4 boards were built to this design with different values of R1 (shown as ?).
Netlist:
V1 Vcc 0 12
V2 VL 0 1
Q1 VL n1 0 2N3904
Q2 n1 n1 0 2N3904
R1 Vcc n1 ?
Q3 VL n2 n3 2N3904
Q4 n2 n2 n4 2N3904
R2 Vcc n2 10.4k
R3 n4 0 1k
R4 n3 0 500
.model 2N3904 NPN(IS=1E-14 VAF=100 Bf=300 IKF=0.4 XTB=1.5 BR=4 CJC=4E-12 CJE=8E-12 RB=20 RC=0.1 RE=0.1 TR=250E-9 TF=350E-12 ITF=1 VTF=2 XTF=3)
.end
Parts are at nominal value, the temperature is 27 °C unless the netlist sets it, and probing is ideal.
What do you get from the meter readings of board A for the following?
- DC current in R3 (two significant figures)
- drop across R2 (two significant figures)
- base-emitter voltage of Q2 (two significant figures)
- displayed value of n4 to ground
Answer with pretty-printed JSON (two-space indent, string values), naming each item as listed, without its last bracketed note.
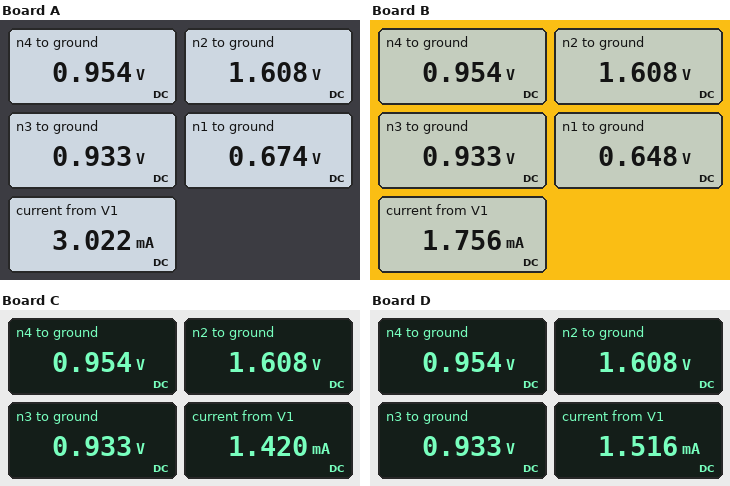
{
  "DC current in R3": "950 µA",
  "drop across R2": "10 V",
  "base-emitter voltage of Q2": "670 mV",
  "displayed value of n4 to ground": "0.954 V"
}
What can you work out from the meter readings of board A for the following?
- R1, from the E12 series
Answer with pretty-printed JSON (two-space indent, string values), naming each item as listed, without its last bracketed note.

{
  "R1, from the E12 series": "5.6 kΩ"
}
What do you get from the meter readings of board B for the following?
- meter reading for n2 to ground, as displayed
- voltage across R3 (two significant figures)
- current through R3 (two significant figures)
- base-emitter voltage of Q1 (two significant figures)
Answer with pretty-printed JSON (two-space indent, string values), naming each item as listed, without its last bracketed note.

{
  "meter reading for n2 to ground, as displayed": "1.608 V",
  "voltage across R3": "950 mV",
  "current through R3": "950 µA",
  "base-emitter voltage of Q1": "650 mV"
}
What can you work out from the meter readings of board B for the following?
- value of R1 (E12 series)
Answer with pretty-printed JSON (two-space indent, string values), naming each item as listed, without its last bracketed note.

{
  "value of R1": "15 kΩ"
}
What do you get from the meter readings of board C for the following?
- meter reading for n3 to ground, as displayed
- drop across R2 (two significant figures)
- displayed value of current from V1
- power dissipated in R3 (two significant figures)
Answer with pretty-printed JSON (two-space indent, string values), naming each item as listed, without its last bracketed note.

{
  "meter reading for n3 to ground, as displayed": "0.933 V",
  "drop across R2": "10 V",
  "displayed value of current from V1": "1.420 mA",
  "power dissipated in R3": "910 µW"
}
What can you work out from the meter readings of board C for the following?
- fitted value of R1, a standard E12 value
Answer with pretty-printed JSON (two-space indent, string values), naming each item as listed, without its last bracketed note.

{
  "fitted value of R1, a standard E12 value": "27 kΩ"
}
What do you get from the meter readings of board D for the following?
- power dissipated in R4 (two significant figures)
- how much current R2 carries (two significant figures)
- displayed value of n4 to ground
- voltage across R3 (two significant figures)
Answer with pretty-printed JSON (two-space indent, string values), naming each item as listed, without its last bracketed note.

{
  "power dissipated in R4": "1.7 mW",
  "how much current R2 carries": "1.0 mA",
  "displayed value of n4 to ground": "0.954 V",
  "voltage across R3": "950 mV"
}
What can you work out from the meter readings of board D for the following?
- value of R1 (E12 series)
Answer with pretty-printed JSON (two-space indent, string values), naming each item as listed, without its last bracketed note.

{
  "value of R1": "22 kΩ"
}
